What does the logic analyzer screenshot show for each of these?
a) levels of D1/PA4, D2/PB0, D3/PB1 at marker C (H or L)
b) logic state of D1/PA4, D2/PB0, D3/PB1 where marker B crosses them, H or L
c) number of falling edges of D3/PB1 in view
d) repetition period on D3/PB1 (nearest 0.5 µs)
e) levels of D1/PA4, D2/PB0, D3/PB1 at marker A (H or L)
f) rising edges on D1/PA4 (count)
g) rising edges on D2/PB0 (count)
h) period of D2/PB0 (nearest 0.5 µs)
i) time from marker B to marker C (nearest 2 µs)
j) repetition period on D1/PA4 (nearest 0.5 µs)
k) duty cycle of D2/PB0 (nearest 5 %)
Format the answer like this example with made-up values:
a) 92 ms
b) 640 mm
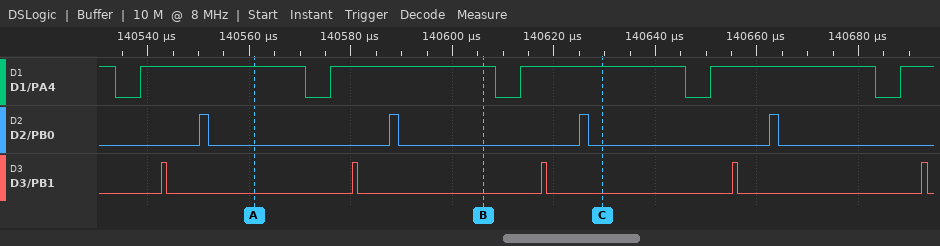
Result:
a) D1/PA4=H, D2/PB0=L, D3/PB1=L
b) D1/PA4=H, D2/PB0=L, D3/PB1=L
c) 5
d) 37.5 µs
e) D1/PA4=H, D2/PB0=L, D3/PB1=L
f) 5
g) 4
h) 37.5 µs
i) 24 µs
j) 37.5 µs
k) 5 %
